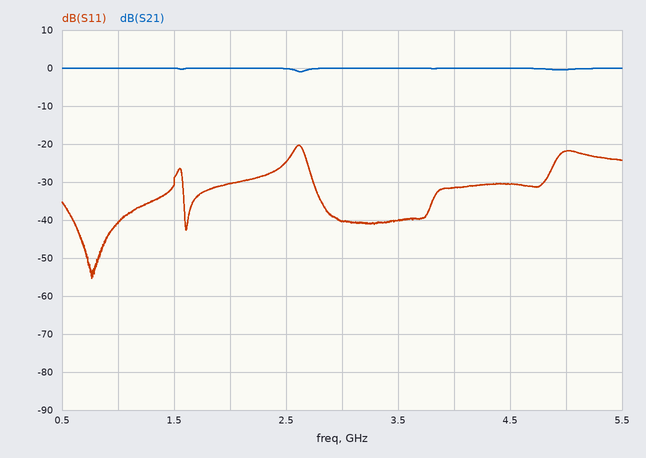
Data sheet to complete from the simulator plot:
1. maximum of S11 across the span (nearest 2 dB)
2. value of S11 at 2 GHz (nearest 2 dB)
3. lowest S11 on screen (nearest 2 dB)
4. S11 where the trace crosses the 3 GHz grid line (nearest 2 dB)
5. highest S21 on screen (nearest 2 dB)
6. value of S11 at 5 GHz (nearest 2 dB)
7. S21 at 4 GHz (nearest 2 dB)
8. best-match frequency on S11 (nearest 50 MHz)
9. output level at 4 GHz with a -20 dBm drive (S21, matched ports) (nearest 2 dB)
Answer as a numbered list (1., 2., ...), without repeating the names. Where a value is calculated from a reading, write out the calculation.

1. -20 dB
2. -30 dB
3. -56 dB
4. -40 dB
5. 0 dB
6. -22 dB
7. 0 dB
8. 750 MHz
9. -20 dBm + (0 dB) = -20 dBm
